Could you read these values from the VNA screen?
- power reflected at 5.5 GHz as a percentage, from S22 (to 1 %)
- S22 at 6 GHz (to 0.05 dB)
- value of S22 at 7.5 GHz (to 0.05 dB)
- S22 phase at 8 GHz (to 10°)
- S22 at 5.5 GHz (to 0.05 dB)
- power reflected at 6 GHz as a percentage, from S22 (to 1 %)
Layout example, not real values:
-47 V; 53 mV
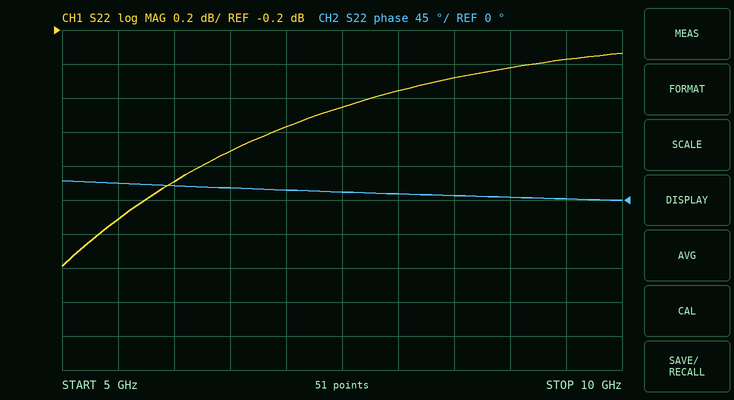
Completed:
74 %; -1.10 dB; -0.65 dB; 10°; -1.30 dB; 78 %
